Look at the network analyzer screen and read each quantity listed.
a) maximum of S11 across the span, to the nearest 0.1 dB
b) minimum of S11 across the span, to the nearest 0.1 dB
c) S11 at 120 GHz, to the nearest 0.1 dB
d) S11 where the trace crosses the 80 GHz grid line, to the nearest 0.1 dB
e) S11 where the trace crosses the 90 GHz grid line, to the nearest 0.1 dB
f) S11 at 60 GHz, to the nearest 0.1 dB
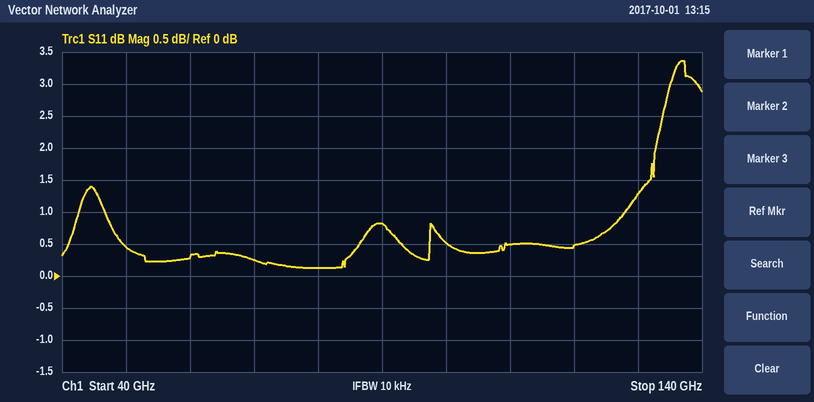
3.4 dB
0.1 dB
0.5 dB
0.1 dB
0.8 dB
0.3 dB
